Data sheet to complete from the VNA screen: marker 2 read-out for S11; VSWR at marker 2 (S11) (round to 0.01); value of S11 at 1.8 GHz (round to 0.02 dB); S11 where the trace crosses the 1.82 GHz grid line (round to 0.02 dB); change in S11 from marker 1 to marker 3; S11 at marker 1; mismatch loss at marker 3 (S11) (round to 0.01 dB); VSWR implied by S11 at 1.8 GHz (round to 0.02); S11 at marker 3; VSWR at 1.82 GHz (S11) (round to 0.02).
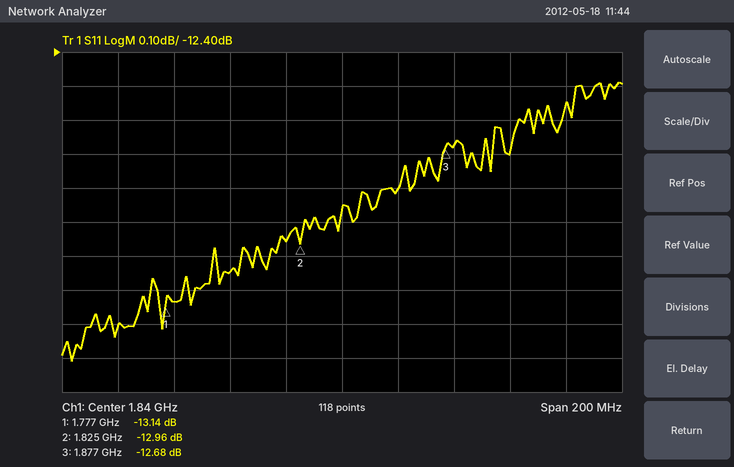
-12.96 dB
1.58
-13.04 dB
-12.96 dB
0.46 dB
-13.14 dB
0.24 dB
1.58
-12.68 dB
1.58
